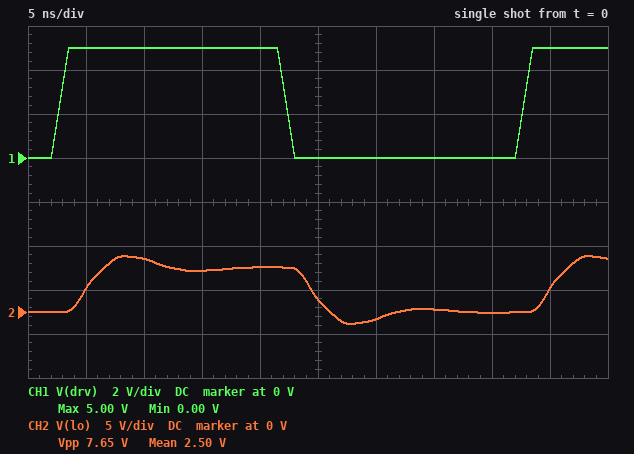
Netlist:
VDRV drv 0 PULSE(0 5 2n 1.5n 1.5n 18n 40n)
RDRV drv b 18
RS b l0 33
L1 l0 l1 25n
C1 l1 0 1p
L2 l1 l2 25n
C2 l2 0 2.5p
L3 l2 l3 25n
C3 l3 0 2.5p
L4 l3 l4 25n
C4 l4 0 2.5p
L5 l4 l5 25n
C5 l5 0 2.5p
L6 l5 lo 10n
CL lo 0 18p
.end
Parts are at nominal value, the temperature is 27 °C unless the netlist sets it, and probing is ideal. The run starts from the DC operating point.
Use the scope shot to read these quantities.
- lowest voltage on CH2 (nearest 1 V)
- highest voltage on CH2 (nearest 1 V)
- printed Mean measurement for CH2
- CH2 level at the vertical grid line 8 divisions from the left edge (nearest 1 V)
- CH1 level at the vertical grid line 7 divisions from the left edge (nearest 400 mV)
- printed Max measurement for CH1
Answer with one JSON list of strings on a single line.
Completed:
["-1 V", "6 V", "2.50 V", "0 V", "0 V", "5.00 V"]
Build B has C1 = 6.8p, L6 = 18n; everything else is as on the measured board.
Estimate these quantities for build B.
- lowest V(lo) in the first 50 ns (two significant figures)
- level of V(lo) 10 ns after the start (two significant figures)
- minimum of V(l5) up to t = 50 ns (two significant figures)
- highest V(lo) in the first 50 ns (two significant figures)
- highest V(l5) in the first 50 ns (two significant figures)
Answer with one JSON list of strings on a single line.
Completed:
["-1.2 V", "5.9 V", "-1.1 V", "6.2 V", "6.1 V"]
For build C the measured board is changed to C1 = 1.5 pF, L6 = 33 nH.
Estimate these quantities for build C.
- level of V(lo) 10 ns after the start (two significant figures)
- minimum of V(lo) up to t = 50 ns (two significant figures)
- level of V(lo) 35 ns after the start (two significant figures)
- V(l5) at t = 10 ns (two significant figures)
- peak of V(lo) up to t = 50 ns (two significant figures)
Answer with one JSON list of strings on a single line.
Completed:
["6.2 V", "-1.6 V", "400 mV", "6.3 V", "6.6 V"]
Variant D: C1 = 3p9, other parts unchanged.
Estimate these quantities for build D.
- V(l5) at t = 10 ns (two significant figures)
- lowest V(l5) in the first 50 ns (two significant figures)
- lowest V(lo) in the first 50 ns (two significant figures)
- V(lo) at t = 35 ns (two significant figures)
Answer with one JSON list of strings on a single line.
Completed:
["5.9 V", "-1.2 V", "-1.3 V", "240 mV"]
